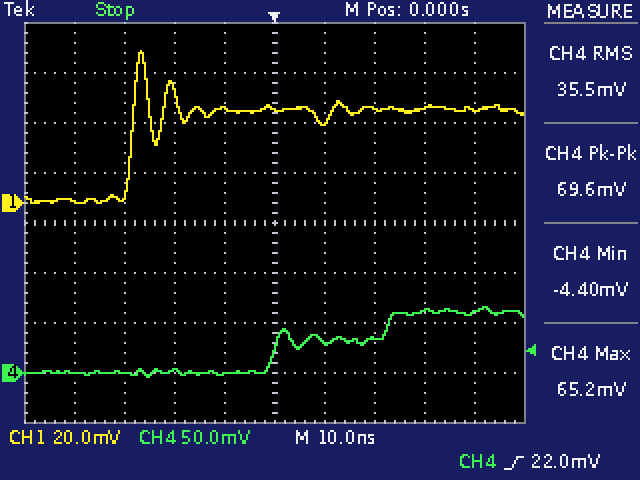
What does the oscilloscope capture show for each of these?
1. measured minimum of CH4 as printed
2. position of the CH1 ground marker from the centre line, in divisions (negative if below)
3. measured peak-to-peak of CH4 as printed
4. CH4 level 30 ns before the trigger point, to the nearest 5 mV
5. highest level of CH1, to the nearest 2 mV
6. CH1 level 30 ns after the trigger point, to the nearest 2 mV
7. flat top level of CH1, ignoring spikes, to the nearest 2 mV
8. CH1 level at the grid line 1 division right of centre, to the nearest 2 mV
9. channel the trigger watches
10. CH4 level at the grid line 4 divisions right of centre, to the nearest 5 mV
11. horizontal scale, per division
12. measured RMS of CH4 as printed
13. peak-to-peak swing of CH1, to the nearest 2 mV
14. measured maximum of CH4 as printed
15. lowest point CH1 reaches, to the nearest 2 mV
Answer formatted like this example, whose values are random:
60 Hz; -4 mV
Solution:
-4.40 mV; +0.4 div; 69.6 mV; 0 mV; 60 mV; 38 mV; 38 mV; 32 mV; CH4; 60 mV; 10 ns; 35.5 mV; 60 mV; 65.2 mV; 0 mV
